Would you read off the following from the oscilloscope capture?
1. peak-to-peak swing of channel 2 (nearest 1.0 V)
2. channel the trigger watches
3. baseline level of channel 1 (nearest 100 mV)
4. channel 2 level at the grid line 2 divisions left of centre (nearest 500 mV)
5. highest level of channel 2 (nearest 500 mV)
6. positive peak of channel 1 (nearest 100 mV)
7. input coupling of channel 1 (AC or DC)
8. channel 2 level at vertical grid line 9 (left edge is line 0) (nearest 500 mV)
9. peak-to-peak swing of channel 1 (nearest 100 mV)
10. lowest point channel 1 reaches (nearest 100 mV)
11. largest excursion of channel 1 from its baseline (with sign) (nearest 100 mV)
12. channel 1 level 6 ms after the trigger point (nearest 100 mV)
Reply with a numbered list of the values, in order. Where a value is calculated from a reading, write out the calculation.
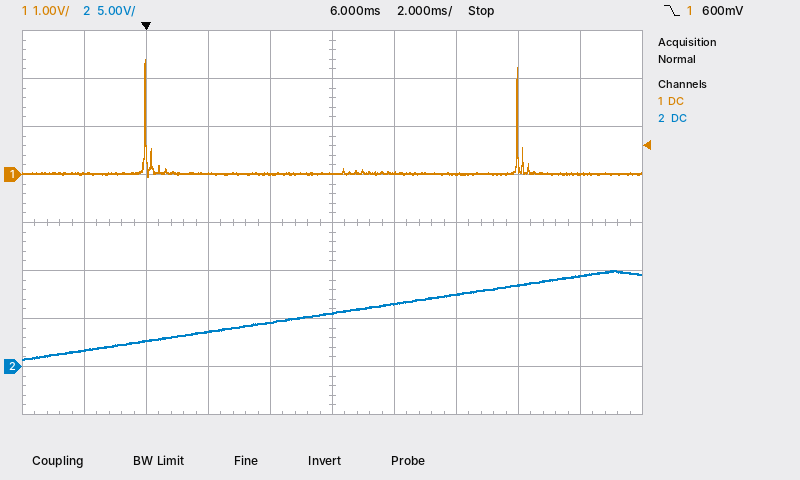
1. 9.0 V
2. channel 1
3. 0.0 V
4. 3.5 V
5. 10.0 V
6. 2.4 V
7. DC
8. 9.5 V
9. 2.4 V − (0.0 V) = 2.4 V
10. 0.0 V
11. 2.4 V − (0.0 V) = +2.4 V
12. 0.0 V
